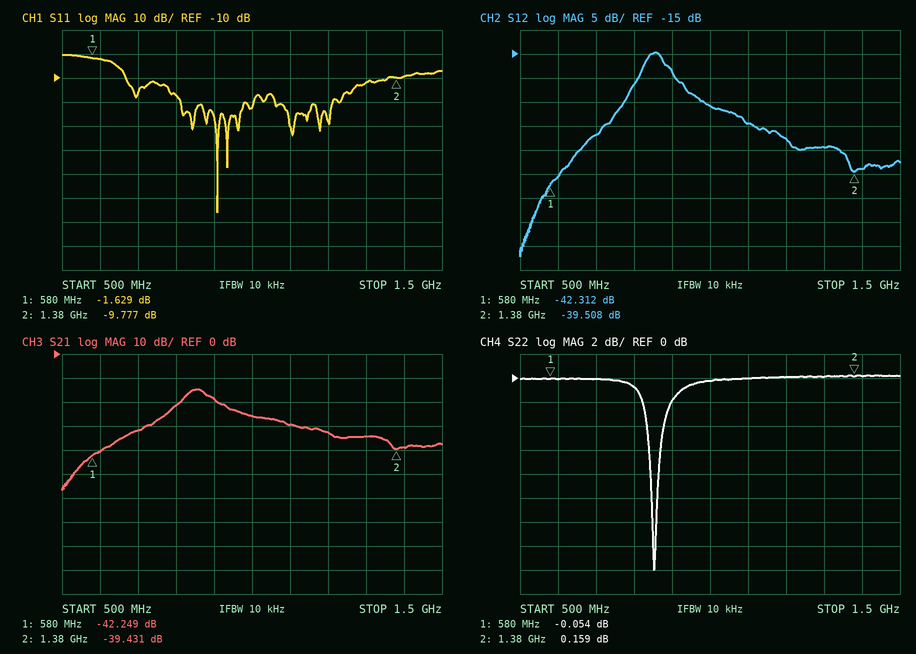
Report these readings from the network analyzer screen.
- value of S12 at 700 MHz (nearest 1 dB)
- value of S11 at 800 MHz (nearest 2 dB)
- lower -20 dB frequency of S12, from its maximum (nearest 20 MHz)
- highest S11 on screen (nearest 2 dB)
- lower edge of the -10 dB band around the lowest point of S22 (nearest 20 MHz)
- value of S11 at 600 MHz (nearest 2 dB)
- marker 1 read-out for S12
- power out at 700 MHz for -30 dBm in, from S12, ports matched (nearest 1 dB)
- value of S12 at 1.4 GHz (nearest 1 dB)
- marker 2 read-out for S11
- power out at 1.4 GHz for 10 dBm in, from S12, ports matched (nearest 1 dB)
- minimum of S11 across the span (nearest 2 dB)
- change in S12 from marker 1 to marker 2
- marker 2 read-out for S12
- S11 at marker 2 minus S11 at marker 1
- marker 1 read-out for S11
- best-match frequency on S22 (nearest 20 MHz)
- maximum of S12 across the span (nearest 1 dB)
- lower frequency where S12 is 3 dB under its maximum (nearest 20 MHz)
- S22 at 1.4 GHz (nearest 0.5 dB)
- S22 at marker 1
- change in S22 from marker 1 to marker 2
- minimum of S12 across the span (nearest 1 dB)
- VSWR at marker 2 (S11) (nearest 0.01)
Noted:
-32 dB
-18 dB
660 MHz
0 dB
840 MHz
-2 dB
-42.312 dB
-62 dBm
-39 dB
-9.777 dB
-29 dBm
-66 dB
2.804 dB
-39.508 dB
-8.148 dB
-1.629 dB
860 MHz
-15 dB
820 MHz
0.0 dB
-0.054 dB
0.213 dB
-57 dB
1.96
